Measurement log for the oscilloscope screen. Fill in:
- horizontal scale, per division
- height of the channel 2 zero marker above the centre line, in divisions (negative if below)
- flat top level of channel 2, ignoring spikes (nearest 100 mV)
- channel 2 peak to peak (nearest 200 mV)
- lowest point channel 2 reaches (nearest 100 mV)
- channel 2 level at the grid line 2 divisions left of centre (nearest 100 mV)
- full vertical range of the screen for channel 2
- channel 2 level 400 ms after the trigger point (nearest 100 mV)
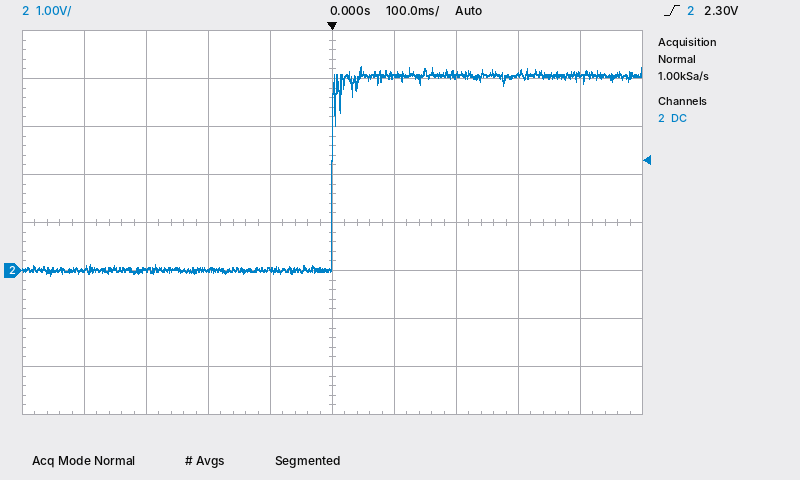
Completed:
100 ms
-1.0 div
4.1 V
4.4 V
-100 mV
0.0 V
8 V
4.1 V
